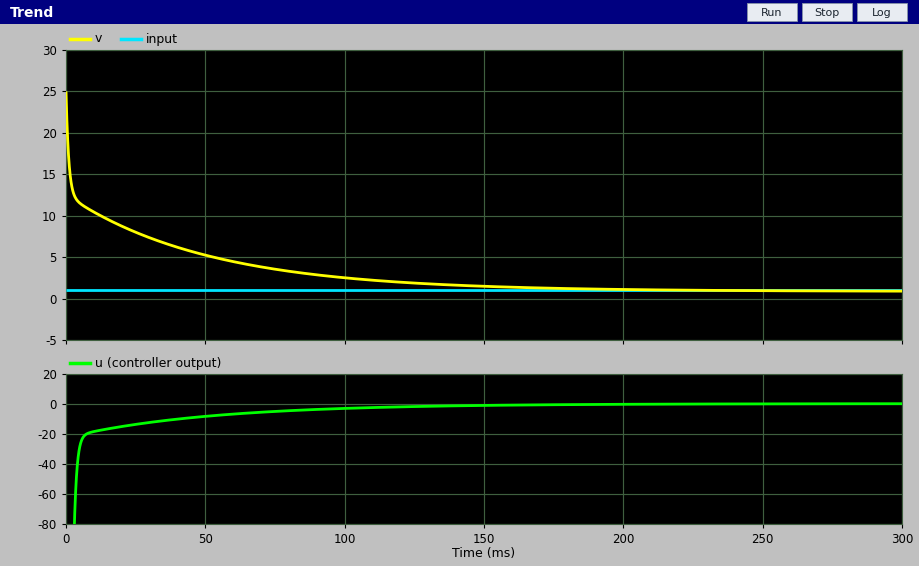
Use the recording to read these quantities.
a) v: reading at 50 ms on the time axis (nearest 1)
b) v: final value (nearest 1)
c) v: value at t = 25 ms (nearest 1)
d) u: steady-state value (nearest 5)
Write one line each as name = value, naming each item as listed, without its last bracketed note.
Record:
v: reading at 50 ms on the time axis = 5
v: final value = 1
v: value at t = 25 ms = 8
u: steady-state value = 0
